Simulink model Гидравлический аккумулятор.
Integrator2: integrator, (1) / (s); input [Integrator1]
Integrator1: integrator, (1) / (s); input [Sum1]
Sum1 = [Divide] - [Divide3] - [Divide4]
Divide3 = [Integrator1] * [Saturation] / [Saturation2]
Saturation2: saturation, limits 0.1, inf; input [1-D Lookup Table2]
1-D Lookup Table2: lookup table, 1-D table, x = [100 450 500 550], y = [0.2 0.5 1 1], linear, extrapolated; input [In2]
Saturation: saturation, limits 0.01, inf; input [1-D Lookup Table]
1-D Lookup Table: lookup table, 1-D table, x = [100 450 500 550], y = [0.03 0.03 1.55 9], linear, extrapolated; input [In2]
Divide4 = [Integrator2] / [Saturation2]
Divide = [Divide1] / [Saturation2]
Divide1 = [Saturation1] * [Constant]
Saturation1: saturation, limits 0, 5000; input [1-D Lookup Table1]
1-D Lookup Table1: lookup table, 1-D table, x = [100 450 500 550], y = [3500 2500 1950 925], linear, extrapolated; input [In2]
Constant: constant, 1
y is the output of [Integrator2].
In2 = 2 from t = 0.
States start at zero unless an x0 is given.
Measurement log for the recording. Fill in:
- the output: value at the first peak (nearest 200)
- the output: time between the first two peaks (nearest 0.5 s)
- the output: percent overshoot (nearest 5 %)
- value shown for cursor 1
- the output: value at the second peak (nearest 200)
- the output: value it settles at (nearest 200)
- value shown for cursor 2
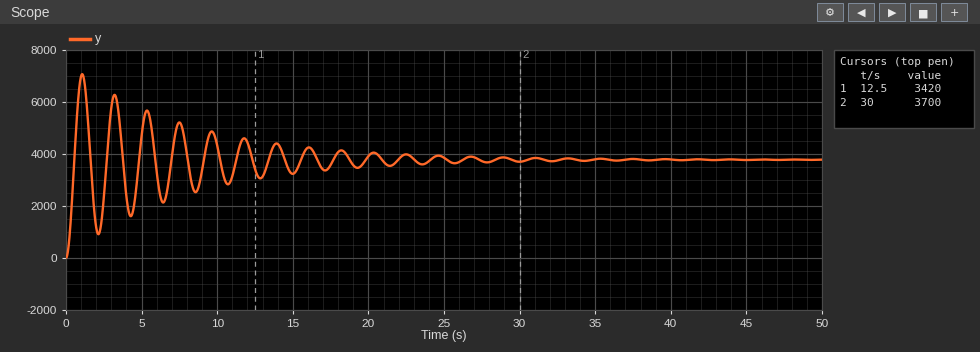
7000
2.0 s
85 %
3420
6200
3800
3700
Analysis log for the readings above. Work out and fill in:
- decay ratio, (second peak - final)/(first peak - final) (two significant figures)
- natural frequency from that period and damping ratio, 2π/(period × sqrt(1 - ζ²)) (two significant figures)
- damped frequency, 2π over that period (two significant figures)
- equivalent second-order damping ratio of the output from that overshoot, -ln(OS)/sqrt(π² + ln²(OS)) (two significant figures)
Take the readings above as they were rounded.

0.75
3.1 rad/s
3.1 rad/s
0.052
